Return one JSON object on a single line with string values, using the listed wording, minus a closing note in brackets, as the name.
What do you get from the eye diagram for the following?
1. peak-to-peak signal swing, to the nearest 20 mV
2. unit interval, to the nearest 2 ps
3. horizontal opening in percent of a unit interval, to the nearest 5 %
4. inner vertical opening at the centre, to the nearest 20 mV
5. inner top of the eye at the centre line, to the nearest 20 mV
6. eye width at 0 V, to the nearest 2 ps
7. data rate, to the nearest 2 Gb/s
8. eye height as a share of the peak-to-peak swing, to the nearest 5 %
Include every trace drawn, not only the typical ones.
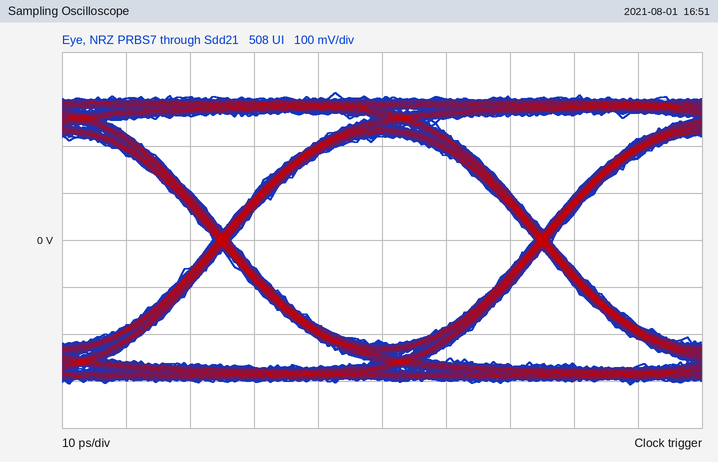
{"peak-to-peak signal swing, to the nearest 20 mV": "620 mV", "unit interval, to the nearest 2 ps": "50 ps", "horizontal opening in percent of a unit interval, to the nearest 5 %": "95 %", "inner vertical opening at the centre, to the nearest 20 mV": "440 mV", "inner top of the eye at the centre line, to the nearest 20 mV": "220 mV", "eye width at 0 V, to the nearest 2 ps": "48 ps", "data rate, to the nearest 2 Gb/s": "20 Gb/s", "eye height as a share of the peak-to-peak swing, to the nearest 5 %": "70 %"}
